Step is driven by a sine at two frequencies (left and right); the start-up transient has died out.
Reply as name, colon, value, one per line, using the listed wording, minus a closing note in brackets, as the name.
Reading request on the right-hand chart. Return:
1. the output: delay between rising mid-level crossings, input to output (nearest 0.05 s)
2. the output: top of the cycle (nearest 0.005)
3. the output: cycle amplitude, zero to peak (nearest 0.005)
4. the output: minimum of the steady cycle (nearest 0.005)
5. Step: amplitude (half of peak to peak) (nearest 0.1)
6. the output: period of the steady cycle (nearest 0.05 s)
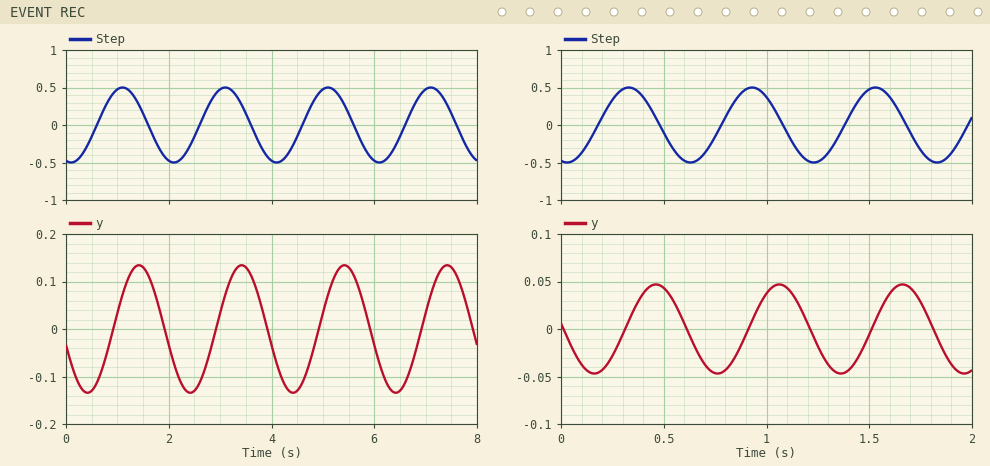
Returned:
the output: delay between rising mid-level crossings, input to output: 0.15 s
the output: top of the cycle: 0.045
the output: cycle amplitude, zero to peak: 0.045
the output: minimum of the steady cycle: -0.045
Step: amplitude (half of peak to peak): 0.5
the output: period of the steady cycle: 0.60 s
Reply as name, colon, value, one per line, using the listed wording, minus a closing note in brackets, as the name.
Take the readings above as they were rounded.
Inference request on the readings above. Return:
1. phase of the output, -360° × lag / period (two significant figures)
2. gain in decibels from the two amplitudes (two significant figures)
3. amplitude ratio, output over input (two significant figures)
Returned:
phase of the output, -360° × lag / period: -90°
gain in decibels from the two amplitudes: -21 dB
amplitude ratio, output over input: 0.090
